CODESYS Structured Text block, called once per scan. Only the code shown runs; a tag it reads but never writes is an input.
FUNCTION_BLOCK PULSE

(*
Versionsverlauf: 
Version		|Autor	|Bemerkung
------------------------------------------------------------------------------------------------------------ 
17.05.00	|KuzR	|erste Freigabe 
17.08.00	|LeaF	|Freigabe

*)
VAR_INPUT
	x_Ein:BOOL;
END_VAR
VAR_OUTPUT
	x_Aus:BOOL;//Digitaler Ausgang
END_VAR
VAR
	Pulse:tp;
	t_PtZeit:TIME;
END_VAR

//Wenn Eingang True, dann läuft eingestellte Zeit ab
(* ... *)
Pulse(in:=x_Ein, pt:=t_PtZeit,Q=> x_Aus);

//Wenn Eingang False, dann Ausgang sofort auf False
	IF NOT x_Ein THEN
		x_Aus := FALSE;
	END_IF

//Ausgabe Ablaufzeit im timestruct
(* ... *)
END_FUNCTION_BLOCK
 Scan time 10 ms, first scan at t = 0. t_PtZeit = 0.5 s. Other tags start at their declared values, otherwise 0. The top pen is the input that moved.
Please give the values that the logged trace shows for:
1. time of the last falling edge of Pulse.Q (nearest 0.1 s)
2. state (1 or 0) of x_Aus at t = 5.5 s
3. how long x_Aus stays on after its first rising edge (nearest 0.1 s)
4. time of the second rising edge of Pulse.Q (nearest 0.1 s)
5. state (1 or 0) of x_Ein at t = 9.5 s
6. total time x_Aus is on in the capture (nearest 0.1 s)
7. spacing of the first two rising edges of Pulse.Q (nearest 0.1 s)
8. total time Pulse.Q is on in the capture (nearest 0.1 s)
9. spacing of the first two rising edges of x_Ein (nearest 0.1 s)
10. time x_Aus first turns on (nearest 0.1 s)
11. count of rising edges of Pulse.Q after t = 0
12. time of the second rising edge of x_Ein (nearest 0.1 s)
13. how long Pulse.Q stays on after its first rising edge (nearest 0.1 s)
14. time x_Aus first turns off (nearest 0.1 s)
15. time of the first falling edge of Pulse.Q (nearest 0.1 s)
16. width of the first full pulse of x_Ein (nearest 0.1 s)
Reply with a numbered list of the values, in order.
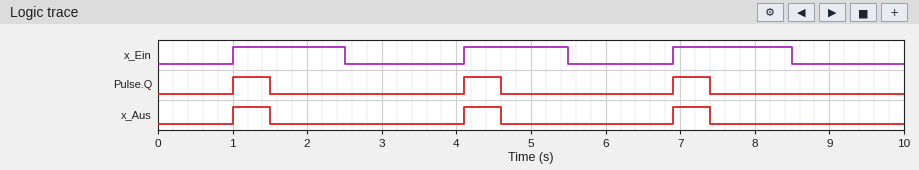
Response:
1. 7.4 s
2. 0
3. 0.5 s
4. 4.1 s
5. 0
6. 1.5 s
7. 3.1 s
8. 1.5 s
9. 3.1 s
10. 1.0 s
11. 3
12. 4.1 s
13. 0.5 s
14. 1.5 s
15. 1.5 s
16. 1.5 s
